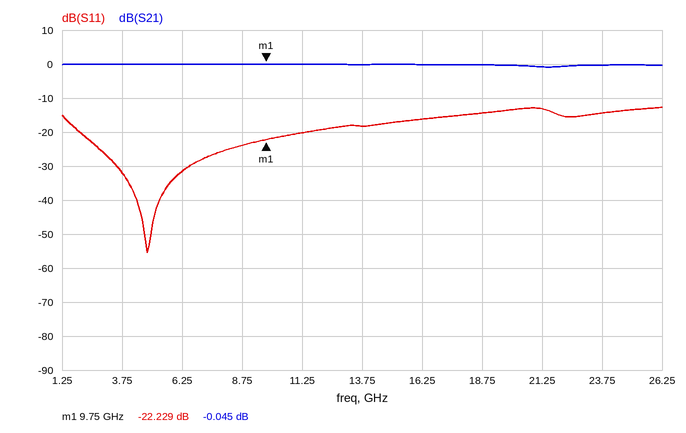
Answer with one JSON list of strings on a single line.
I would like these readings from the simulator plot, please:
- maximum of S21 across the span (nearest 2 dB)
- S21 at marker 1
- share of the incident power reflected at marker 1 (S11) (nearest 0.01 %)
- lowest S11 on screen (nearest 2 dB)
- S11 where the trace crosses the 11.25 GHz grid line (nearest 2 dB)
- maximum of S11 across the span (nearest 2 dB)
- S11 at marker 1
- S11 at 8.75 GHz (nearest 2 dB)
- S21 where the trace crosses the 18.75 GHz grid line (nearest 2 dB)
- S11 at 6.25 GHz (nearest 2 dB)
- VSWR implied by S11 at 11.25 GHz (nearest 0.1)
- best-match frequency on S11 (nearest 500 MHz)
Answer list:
["0 dB", "-0.045 dB", "0.60 %", "-56 dB", "-20 dB", "-12 dB", "-22.229 dB", "-24 dB", "0 dB", "-32 dB", "1.2", "5.0 GHz"]
